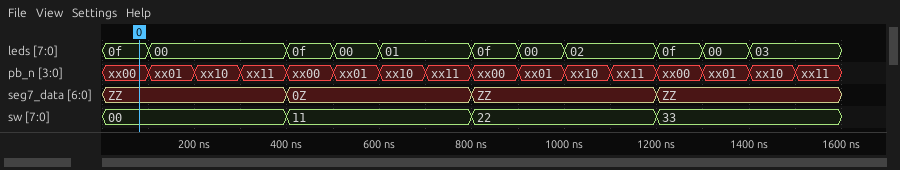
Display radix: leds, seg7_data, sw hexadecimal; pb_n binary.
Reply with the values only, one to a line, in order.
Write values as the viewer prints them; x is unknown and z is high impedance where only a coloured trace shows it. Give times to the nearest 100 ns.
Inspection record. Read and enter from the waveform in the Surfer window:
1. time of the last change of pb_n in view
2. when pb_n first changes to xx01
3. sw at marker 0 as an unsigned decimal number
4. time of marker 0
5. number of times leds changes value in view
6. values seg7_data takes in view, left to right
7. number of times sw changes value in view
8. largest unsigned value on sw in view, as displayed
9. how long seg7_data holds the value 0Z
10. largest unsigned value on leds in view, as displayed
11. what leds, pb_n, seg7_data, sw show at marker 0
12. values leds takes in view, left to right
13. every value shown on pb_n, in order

1500 ns
100 ns
0
100 ns
10
ZZ, 0Z, ZZ, ZZ
3
33
400 ns
0f
leds=0f, pb_n=xx00, seg7_data=ZZ, sw=00
0f, 00, 0f, 00, 01, 0f, 00, 02, 0f, 00, 03
xx00, xx01, xx10, xx11, xx00, xx01, xx10, xx11, xx00, xx01, xx10, xx11, xx00, xx01, xx10, xx11
